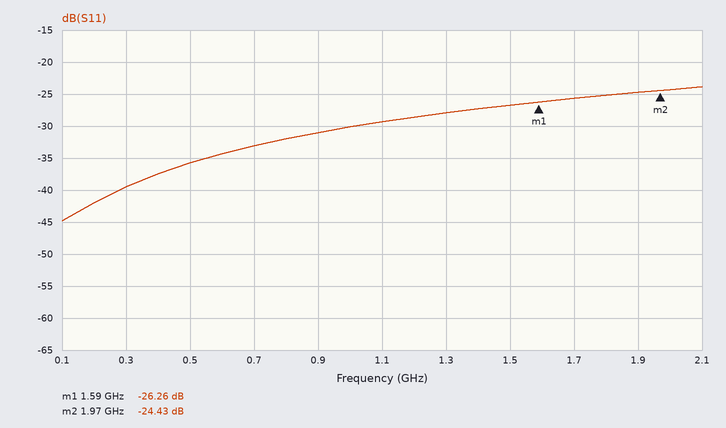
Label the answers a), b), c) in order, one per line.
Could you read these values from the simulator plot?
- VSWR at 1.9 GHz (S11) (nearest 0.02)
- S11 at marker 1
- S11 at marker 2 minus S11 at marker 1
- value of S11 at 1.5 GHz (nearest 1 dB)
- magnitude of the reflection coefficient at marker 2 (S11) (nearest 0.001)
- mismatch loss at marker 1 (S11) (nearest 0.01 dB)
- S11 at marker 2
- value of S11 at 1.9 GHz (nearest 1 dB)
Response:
a) 1.12
b) -26.26 dB
c) 1.83 dB
d) -27 dB
e) 0.060
f) 0.01 dB
g) -24.43 dB
h) -25 dB
